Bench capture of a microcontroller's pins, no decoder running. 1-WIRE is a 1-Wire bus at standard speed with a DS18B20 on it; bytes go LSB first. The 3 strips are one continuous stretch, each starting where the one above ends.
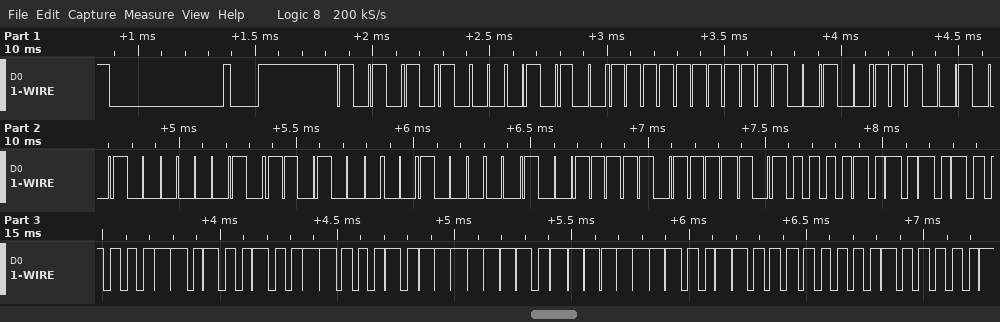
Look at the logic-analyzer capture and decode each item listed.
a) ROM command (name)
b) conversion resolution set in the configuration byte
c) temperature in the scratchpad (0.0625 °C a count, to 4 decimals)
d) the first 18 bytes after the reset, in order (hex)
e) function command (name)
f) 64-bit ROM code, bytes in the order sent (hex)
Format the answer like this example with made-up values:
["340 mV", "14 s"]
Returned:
["Match ROM", "12 bits", "85.0000 °C", "55 28 FF 27 27 81 16 04 F9 BE 50 05 4B 46 7F FF 0C 10", "Read Scratchpad", "28 FF 27 27 81 16 04 F9"]
